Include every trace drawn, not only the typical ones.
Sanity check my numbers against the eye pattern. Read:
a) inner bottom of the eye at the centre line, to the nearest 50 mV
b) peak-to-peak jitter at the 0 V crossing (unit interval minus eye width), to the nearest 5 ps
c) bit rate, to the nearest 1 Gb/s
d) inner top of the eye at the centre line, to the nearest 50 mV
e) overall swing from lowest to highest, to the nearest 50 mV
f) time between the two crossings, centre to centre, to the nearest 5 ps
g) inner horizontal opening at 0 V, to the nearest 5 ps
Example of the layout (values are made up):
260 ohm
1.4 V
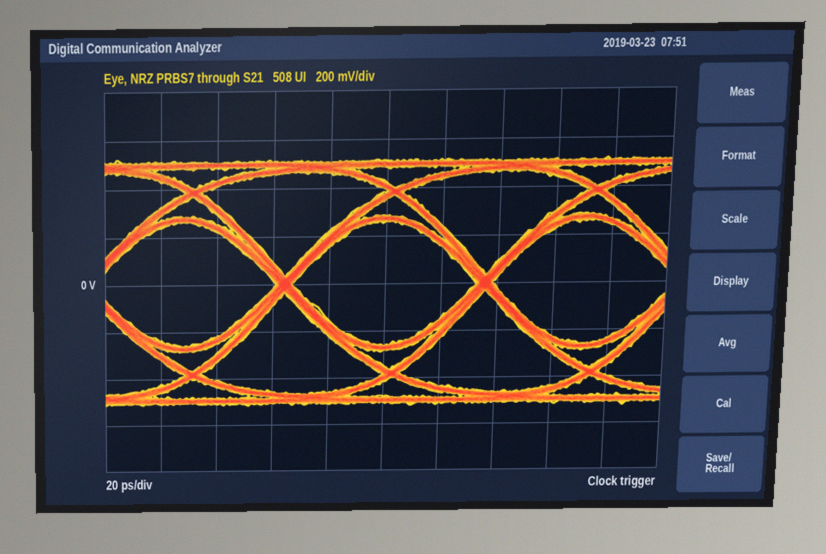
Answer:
-250 mV
5 ps
14 Gb/s
250 mV
1.05 V
70 ps
65 ps
